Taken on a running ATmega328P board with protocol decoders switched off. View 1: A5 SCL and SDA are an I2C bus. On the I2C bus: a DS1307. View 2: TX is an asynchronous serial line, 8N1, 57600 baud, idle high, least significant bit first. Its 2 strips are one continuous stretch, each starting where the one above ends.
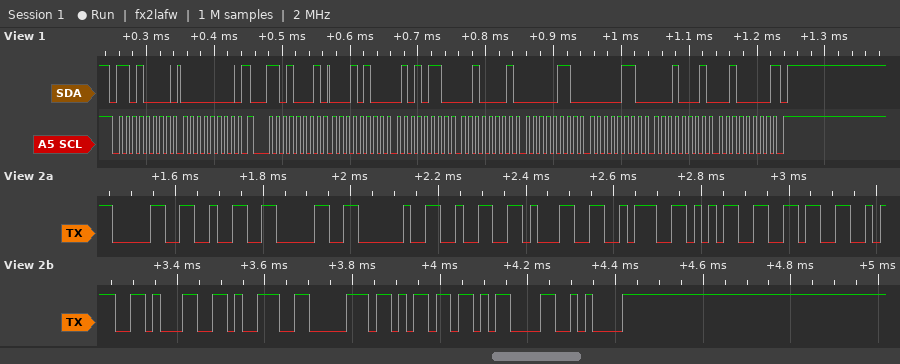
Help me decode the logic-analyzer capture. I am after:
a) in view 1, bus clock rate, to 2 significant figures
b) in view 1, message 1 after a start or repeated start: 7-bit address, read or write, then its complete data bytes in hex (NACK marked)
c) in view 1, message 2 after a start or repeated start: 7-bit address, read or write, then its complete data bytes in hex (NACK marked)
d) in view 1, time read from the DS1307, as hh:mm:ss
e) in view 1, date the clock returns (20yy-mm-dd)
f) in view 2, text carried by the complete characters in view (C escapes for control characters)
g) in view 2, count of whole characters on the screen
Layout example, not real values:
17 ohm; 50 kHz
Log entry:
100 kHz; 0x68 write: 00; 0x68 read: 14 56 21 06 06 11 20 NACK; 21:56:14; 2020-11-06; "020 21:56:19pm\r\n"; 16
